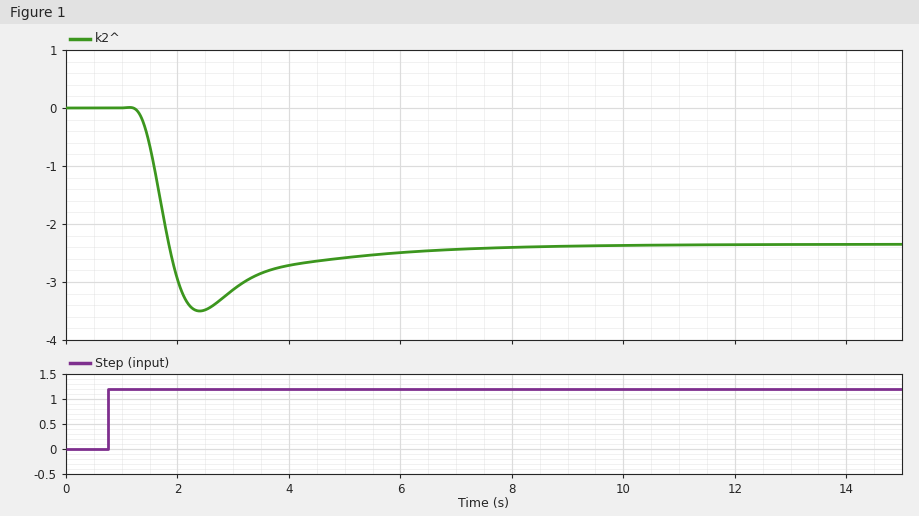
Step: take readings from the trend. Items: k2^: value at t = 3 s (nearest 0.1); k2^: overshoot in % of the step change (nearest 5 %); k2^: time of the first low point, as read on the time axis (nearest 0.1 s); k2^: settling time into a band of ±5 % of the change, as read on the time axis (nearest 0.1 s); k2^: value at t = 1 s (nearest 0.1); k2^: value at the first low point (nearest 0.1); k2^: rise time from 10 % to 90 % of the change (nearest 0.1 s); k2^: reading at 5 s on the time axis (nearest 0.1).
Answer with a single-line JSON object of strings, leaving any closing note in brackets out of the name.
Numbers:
{"k2^: value at t = 3 s": "-3.1", "k2^: overshoot in % of the step change": "50 %", "k2^: time of the first low point, as read on the time axis": "2.4 s", "k2^: settling time into a band of ±5 % of the change, as read on the time axis": "6.4 s", "k2^: value at t = 1 s": "0.0", "k2^: value at the first low point": "-3.5", "k2^: rise time from 10 % to 90 % of the change": "0.4 s", "k2^: reading at 5 s on the time axis": "-2.6"}
